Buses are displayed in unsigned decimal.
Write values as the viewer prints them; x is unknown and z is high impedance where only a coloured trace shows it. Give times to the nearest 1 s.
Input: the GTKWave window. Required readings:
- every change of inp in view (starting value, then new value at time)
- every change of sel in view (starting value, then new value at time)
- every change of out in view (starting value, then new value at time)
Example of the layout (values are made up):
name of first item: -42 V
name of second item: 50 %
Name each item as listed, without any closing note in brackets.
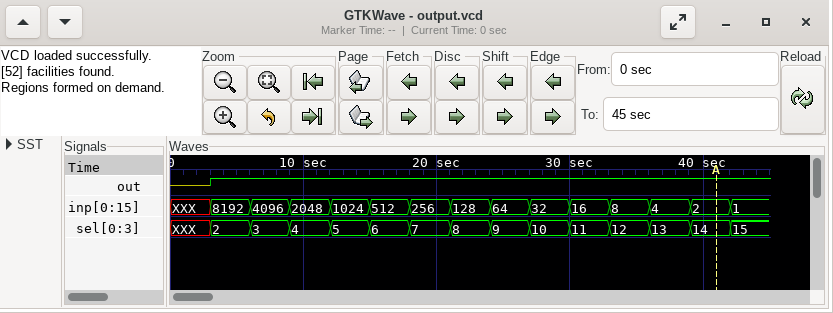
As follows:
every change of inp in view: XXX, 8192 at 3 s, 4096 at 6 s, 2048 at 9 s, 1024 at 12 s, 512 at 15 s, 256 at 18 s, 128 at 21 s, 64 at 24 s, 32 at 27 s, 16 at 30 s, 8 at 33 s, 4 at 36 s, 2 at 39 s, 1 at 42 s
every change of sel in view: XXX, 2 at 3 s, 3 at 6 s, 4 at 9 s, 5 at 12 s, 6 at 15 s, 7 at 18 s, 8 at 21 s, 9 at 24 s, 10 at 27 s, 11 at 30 s, 12 at 33 s, 13 at 36 s, 14 at 39 s, 15 at 42 s
every change of out in view: z, 1 at 3 s
